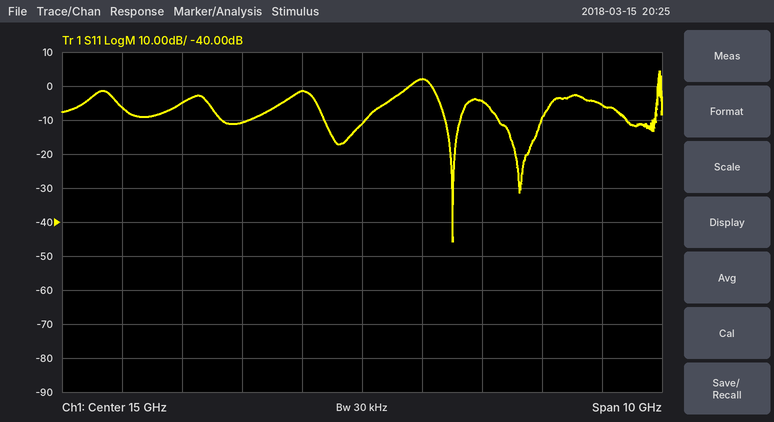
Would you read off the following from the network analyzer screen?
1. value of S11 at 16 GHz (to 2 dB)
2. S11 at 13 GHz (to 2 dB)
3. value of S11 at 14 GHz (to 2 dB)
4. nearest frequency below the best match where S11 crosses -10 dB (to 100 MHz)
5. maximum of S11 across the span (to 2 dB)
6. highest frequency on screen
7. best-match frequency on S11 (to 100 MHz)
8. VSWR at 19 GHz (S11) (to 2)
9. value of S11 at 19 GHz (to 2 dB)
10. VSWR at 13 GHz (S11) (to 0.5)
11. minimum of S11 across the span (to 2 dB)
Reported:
2 dB
-10 dB
-2 dB
16.4 GHz
4 dB
20 GHz
16.5 GHz
4
-6 dB
2.0
-46 dB
